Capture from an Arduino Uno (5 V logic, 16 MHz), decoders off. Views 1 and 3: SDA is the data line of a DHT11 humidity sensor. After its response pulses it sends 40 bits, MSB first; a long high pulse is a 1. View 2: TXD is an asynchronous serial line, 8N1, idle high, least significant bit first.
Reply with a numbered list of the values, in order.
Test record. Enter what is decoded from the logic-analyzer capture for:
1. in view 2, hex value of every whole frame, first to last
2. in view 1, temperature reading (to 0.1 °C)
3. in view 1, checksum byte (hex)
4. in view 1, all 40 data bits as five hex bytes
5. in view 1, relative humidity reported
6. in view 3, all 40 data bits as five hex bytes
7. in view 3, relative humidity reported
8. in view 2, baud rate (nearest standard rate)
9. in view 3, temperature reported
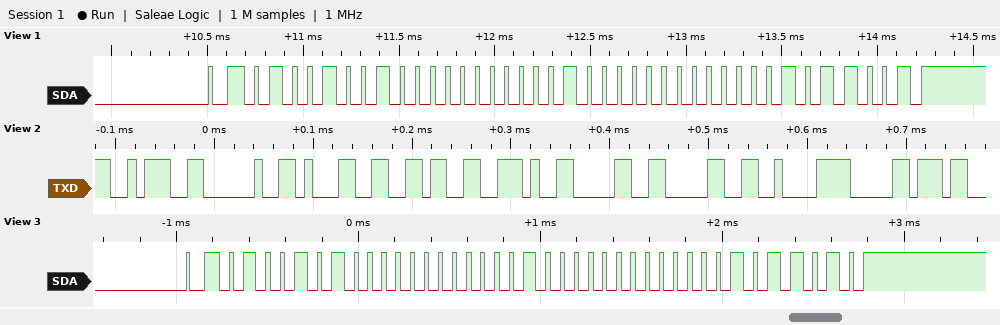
1. 0x3A 0x20 0x31 0x36 0x2E 0x30 0x30 0xC2 0xB0
2. 16.0 °C
3. 0x59
4. 49 00 10 00 59
5. 73 %
6. 4A 00 10 00 5A
7. 74 %
8. 115200 baud
9. 16.0 °C
